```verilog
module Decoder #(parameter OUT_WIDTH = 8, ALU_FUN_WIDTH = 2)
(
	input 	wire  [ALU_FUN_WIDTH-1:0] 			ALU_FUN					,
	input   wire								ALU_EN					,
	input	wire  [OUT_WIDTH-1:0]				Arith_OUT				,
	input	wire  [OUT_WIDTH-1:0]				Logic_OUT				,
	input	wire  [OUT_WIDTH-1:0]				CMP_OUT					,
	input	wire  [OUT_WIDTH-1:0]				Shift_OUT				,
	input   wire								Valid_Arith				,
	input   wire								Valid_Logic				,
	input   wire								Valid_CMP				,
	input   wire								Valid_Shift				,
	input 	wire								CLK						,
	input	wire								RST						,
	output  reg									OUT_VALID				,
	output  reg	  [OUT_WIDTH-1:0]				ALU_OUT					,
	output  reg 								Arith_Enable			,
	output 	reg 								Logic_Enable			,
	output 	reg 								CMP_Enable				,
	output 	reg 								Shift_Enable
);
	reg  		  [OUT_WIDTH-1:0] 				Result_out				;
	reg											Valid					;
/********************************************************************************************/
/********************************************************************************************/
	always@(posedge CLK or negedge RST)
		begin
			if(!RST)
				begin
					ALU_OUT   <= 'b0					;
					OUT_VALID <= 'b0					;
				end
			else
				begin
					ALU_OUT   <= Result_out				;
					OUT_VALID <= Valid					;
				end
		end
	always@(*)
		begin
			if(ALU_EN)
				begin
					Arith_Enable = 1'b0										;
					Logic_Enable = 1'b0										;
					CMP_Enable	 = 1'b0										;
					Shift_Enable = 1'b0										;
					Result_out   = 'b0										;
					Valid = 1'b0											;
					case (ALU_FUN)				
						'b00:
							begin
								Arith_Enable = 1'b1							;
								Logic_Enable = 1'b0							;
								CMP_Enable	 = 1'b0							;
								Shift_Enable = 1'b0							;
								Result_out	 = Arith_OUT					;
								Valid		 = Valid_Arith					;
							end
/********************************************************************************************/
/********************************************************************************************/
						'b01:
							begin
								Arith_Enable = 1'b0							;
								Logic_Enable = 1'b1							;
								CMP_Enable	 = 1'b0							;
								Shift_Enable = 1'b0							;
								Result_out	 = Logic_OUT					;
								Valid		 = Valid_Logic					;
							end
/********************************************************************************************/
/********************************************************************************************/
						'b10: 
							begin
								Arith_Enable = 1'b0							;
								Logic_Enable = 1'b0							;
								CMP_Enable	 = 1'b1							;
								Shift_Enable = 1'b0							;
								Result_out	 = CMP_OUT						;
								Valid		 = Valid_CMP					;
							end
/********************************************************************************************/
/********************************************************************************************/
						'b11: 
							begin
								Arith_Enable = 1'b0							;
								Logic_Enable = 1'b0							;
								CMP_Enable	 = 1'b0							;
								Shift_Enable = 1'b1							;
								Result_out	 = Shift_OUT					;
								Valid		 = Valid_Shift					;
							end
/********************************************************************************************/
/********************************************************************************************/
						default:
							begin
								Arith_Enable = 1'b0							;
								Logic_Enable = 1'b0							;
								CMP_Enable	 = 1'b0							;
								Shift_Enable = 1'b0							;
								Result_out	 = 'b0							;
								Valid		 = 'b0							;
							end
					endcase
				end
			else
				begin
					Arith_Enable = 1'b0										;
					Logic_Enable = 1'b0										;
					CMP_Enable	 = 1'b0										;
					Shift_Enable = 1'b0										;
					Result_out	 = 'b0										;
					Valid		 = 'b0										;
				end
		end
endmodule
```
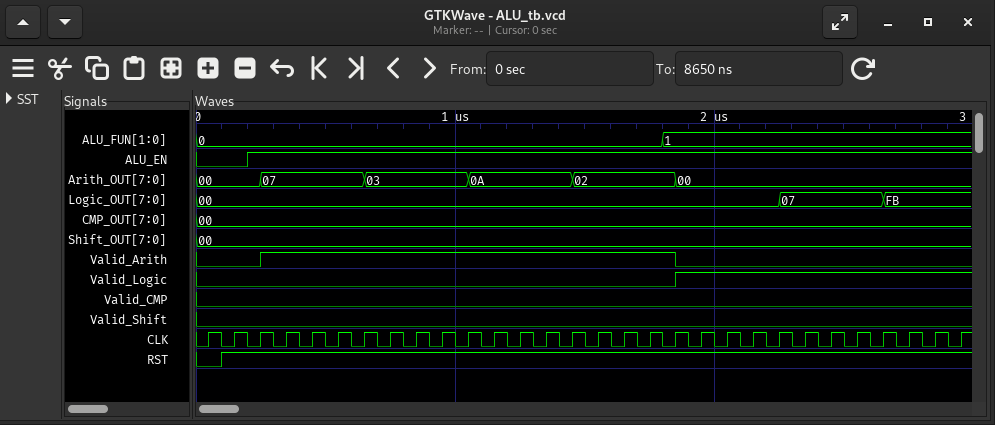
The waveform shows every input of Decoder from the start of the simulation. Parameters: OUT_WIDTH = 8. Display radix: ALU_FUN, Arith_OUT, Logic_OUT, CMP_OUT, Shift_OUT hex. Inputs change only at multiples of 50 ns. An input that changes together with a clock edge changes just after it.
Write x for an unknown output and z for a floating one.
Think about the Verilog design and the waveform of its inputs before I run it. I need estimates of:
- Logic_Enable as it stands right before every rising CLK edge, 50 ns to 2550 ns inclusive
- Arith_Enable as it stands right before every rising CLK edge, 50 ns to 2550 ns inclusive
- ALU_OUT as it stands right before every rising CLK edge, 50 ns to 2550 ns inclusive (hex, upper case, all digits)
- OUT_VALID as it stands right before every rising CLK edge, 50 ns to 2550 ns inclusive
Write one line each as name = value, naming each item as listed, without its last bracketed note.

Logic_Enable as it stands right before every rising CLK edge, 50 ns to 2550 ns inclusive = 0 0 0 0 0 0 0 0 0 0 0 0 0 0 0 0 0 0 1 1 1 1 1 1 1 1
Arith_Enable as it stands right before every rising CLK edge, 50 ns to 2550 ns inclusive = 0 0 1 1 1 1 1 1 1 1 1 1 1 1 1 1 1 1 0 0 0 0 0 0 0 0
ALU_OUT as it stands right before every rising CLK edge, 50 ns to 2550 ns inclusive = 00, 00, 00, 00, 07, 07, 07, 07, 03, 03, 03, 03, 0A, 0A, 0A, 0A, 02, 02, 02, 00, 00, 00, 00, 00, 07, 07
OUT_VALID as it stands right before every rising CLK edge, 50 ns to 2550 ns inclusive = 0 0 0 0 1 1 1 1 1 1 1 1 1 1 1 1 1 1 1 0 1 1 1 1 1 1
